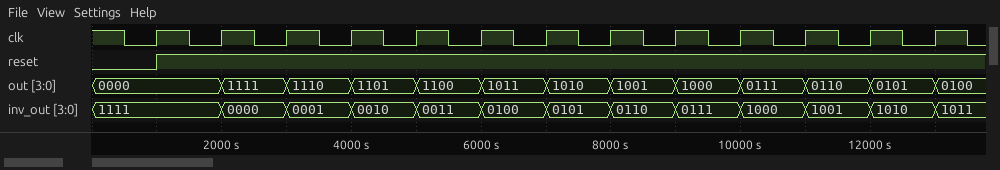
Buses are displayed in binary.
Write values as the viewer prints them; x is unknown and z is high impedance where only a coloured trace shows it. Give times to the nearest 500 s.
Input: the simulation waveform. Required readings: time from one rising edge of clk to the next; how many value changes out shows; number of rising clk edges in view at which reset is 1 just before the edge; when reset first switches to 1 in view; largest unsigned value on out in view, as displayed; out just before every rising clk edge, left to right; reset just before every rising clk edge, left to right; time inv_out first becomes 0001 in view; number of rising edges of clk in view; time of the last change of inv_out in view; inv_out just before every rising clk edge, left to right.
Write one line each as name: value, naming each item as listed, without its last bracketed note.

time from one rising edge of clk to the next: 1000 s
how many value changes out shows: 12
number of rising clk edges in view at which reset is 1 just before the edge: 12
when reset first switches to 1 in view: 1000 s
largest unsigned value on out in view, as displayed: 1111
out just before every rising clk edge, left to right: 0000, 0000, 1111, 1110, 1101, 1100, 1011, 1010, 1001, 1000, 0111, 0110, 0101
reset just before every rising clk edge, left to right: 0 1 1 1 1 1 1 1 1 1 1 1 1
time inv_out first becomes 0001 in view: 3000 s
number of rising edges of clk in view: 13
time of the last change of inv_out in view: 13000 s
inv_out just before every rising clk edge, left to right: 1111, 1111, 0000, 0001, 0010, 0011, 0100, 0101, 0110, 0111, 1000, 1001, 1010
